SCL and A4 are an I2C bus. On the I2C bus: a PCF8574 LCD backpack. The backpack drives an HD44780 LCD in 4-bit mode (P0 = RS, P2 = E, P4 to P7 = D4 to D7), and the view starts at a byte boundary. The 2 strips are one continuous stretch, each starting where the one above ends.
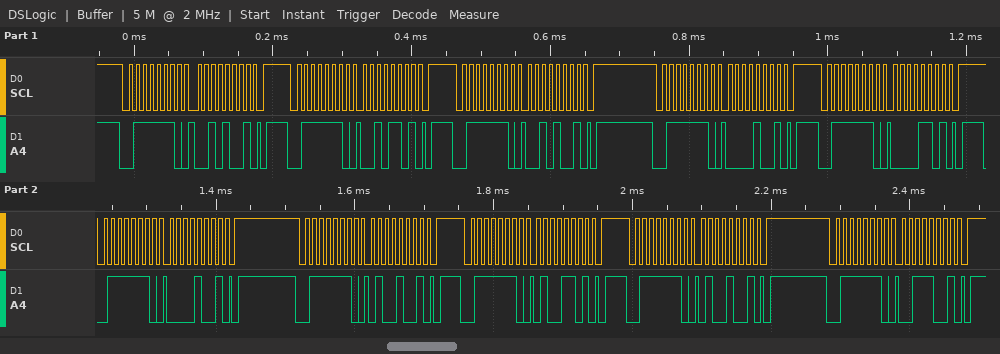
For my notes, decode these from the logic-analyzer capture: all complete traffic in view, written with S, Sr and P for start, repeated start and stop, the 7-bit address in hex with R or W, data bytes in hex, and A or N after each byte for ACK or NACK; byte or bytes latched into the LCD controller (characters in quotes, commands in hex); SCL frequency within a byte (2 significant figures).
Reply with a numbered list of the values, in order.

1. S 3FW A 29 A P S 3FW A 2D A P S 3FW A 29 A P S 3FW A 09 A P S 3FW A 0D A P S 3FW A 09 A P S 3FW A 49 A P S 3FW A 4D A P S 3FW A 49 A P S 3FW A 39 A P
2. ' '
3. 100 kHz
